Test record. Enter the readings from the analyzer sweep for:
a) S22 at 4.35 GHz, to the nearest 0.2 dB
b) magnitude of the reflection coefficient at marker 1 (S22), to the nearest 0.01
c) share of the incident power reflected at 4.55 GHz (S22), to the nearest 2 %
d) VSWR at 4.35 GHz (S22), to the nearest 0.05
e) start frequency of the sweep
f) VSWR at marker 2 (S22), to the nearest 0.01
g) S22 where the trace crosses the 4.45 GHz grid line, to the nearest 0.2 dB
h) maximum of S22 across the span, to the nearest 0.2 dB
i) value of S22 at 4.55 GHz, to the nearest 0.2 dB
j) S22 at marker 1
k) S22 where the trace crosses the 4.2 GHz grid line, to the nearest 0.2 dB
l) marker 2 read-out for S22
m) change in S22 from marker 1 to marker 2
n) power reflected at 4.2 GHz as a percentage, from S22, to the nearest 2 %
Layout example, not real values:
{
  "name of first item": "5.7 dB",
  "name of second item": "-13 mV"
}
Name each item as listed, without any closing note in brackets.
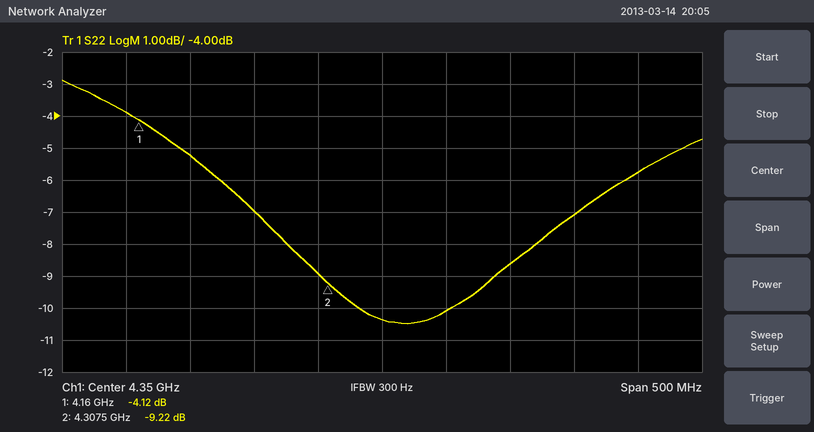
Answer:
{
  "S22 at 4.35 GHz, to the nearest 0.2 dB": "-10.4 dB",
  "magnitude of the reflection coefficient at marker 1 (S22), to the nearest 0.01": "0.62",
  "share of the incident power reflected at 4.55 GHz (S22), to the nearest 2 %": "26 %",
  "VSWR at 4.35 GHz (S22), to the nearest 0.05": "1.85",
  "start frequency of the sweep": "4.1 GHz",
  "VSWR at marker 2 (S22), to the nearest 0.01": "2.06",
  "S22 where the trace crosses the 4.45 GHz grid line, to the nearest 0.2 dB": "-8.6 dB",
  "maximum of S22 across the span, to the nearest 0.2 dB": "-2.8 dB",
  "value of S22 at 4.55 GHz, to the nearest 0.2 dB": "-5.8 dB",
  "S22 at marker 1": "-4.12 dB",
  "S22 where the trace crosses the 4.2 GHz grid line, to the nearest 0.2 dB": "-5.2 dB",
  "marker 2 read-out for S22": "-9.22 dB",
  "change in S22 from marker 1 to marker 2": "-5.10 dB",
  "power reflected at 4.2 GHz as a percentage, from S22, to the nearest 2 %": "30 %"
}
